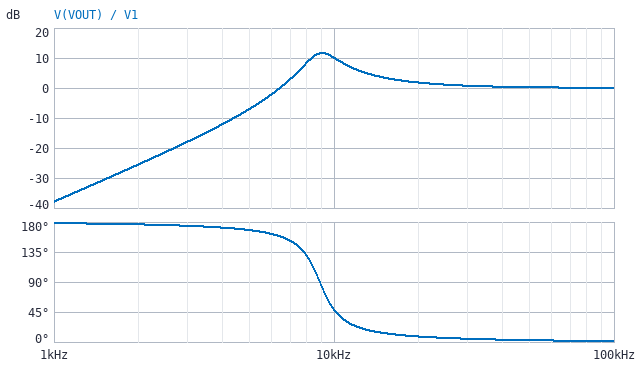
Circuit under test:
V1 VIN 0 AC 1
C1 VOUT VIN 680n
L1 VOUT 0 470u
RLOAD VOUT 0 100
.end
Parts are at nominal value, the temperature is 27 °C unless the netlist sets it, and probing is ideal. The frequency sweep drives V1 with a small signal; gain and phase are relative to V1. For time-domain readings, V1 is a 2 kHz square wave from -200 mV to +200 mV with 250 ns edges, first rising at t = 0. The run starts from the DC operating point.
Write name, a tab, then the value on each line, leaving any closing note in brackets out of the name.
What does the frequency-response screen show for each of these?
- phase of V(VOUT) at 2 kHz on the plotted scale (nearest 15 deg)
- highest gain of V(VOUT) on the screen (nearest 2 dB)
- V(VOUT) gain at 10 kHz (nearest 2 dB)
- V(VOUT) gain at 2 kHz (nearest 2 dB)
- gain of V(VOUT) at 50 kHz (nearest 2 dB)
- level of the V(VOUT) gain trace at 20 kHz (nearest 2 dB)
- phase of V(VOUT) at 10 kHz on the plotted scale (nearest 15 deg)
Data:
phase of V(VOUT) at 2 kHz on the plotted scale	180 deg
highest gain of V(VOUT) on the screen	12 dB
V(VOUT) gain at 10 kHz	10 dB
V(VOUT) gain at 2 kHz	-26 dB
gain of V(VOUT) at 50 kHz	0 dB
level of the V(VOUT) gain trace at 20 kHz	2 dB
phase of V(VOUT) at 10 kHz on the plotted scale	45 deg
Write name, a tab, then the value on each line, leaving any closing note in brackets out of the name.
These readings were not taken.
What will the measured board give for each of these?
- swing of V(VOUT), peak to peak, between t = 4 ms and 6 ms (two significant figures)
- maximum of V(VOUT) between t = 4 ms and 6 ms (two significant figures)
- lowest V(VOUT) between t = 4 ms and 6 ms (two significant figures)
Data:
swing of V(VOUT), peak to peak, between t = 4 ms and 6 ms	760 mV
maximum of V(VOUT) between t = 4 ms and 6 ms	380 mV
lowest V(VOUT) between t = 4 ms and 6 ms	-380 mV
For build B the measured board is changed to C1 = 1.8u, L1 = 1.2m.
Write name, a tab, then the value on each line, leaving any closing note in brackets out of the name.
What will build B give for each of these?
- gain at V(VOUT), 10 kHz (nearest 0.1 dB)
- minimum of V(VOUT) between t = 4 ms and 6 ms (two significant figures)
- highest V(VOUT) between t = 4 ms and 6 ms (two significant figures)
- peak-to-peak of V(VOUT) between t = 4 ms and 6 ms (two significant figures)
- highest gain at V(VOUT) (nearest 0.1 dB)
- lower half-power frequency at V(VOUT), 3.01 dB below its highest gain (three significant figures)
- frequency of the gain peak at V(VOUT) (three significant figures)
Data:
gain at V(VOUT), 10 kHz	1.0 dB
minimum of V(VOUT) between t = 4 ms and 6 ms	-270 mV
highest V(VOUT) between t = 4 ms and 6 ms	270 mV
peak-to-peak of V(VOUT) between t = 4 ms and 6 ms	540 mV
highest gain at V(VOUT)	11.8 dB
lower half-power frequency at V(VOUT), 3.01 dB below its highest gain	3.10 kHz
frequency of the gain peak at V(VOUT)	3.48 kHz
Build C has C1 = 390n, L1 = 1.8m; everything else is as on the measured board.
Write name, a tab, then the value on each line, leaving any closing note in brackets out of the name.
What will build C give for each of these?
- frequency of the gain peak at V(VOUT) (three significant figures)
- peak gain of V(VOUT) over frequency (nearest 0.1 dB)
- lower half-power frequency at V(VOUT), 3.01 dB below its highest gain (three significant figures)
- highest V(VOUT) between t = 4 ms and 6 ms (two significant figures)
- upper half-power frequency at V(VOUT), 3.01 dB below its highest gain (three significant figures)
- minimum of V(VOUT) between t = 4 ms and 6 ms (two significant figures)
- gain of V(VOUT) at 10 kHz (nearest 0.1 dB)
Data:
frequency of the gain peak at V(VOUT)	6.85 kHz
peak gain of V(VOUT) over frequency	3.9 dB
lower half-power frequency at V(VOUT), 3.01 dB below its highest gain	5.06 kHz
highest V(VOUT) between t = 4 ms and 6 ms	420 mV
upper half-power frequency at V(VOUT), 3.01 dB below its highest gain	16.6 kHz
minimum of V(VOUT) between t = 4 ms and 6 ms	-420 mV
gain of V(VOUT) at 10 kHz	2.4 dB
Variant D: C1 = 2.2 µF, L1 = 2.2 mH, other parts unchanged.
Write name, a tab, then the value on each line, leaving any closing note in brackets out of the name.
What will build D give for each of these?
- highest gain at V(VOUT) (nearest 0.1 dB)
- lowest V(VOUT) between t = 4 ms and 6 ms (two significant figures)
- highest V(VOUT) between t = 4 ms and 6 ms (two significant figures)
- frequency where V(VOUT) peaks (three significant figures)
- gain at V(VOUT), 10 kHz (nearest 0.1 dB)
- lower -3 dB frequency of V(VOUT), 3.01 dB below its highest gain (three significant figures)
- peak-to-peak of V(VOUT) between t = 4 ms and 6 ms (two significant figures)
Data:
highest gain at V(VOUT)	10.1 dB
lowest V(VOUT) between t = 4 ms and 6 ms	-630 mV
highest V(VOUT) between t = 4 ms and 6 ms	630 mV
frequency where V(VOUT) peaks	2.35 kHz
gain at V(VOUT), 10 kHz	0.4 dB
lower -3 dB frequency of V(VOUT), 3.01 dB below its highest gain	2.04 kHz
peak-to-peak of V(VOUT) between t = 4 ms and 6 ms	1.3 V
